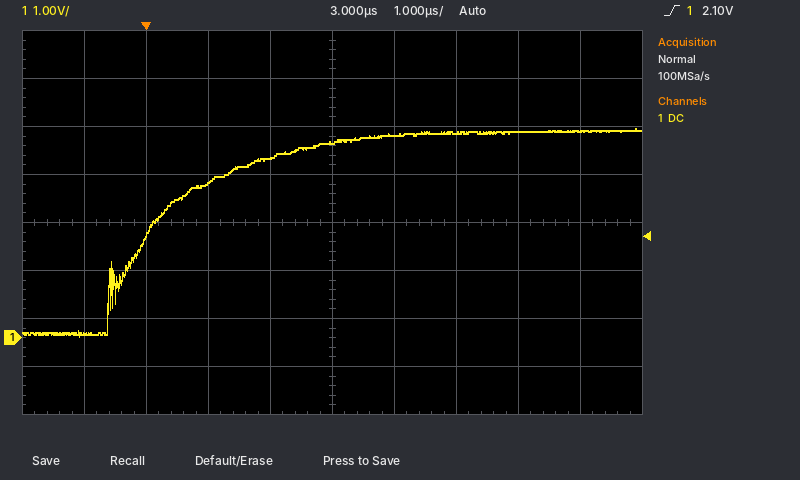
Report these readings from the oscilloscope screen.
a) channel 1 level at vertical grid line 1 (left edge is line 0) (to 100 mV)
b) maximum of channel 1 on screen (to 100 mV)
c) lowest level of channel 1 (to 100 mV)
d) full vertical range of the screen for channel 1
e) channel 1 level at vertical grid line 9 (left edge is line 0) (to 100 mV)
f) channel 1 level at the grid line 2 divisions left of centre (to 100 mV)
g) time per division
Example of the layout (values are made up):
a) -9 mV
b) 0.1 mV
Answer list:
a) 100 mV
b) 4.4 V
c) 0.0 V
d) 8 V
e) 4.3 V
f) 3.2 V
g) 1 µs
